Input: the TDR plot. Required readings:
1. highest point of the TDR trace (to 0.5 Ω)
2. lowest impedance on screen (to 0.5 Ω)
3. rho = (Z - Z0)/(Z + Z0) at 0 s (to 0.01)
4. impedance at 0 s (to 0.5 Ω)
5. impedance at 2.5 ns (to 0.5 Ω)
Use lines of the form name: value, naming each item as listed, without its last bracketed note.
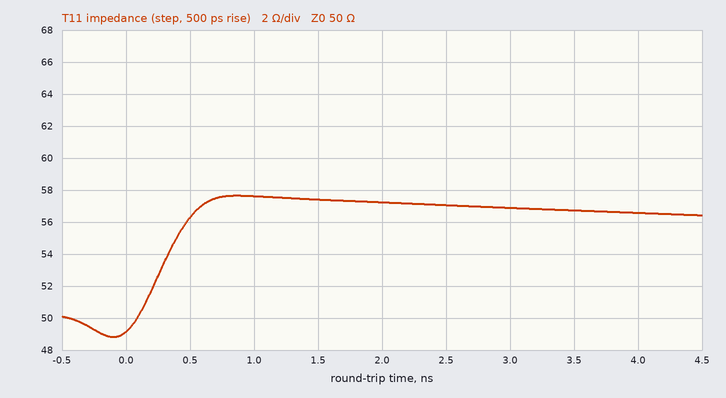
highest point of the TDR trace: 57.5 Ω
lowest impedance on screen: 49.0 Ω
rho = (Z - Z0)/(Z + Z0) at 0 s: -0.01
impedance at 0 s: 49.0 Ω
impedance at 2.5 ns: 57.0 Ω
